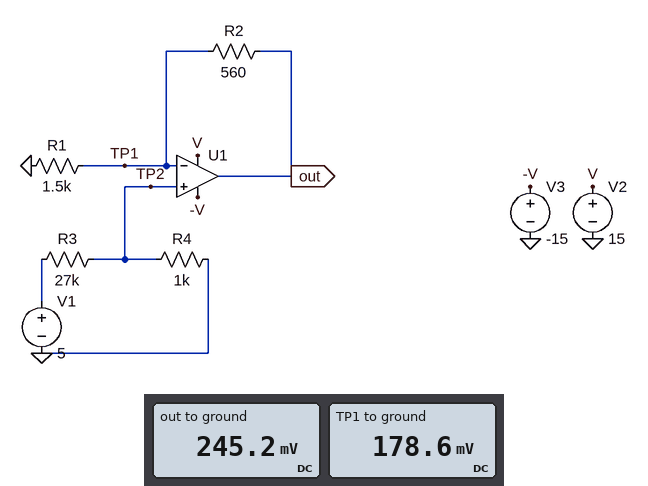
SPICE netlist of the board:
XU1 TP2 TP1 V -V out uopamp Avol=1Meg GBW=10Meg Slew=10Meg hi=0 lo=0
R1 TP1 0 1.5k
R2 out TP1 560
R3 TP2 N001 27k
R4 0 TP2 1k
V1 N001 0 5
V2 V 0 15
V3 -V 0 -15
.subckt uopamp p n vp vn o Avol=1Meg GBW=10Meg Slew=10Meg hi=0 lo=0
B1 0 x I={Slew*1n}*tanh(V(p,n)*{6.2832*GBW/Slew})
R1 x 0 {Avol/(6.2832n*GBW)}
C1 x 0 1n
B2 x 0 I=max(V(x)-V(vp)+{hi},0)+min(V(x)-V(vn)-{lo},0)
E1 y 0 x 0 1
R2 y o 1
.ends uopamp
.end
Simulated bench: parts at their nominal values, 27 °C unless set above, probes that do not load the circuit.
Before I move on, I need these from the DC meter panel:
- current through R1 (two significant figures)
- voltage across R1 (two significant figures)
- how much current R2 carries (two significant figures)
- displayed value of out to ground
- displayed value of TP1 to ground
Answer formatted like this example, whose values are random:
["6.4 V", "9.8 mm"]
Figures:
["120 µA", "180 mV", "120 µA", "245.2 mV", "178.6 mV"]
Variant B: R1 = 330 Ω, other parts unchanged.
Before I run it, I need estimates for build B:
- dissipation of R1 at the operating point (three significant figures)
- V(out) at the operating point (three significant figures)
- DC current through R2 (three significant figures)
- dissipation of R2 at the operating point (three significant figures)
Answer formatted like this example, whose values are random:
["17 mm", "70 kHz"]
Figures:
["96.6 µW", "482 mV", "541 µA", "164 µW"]
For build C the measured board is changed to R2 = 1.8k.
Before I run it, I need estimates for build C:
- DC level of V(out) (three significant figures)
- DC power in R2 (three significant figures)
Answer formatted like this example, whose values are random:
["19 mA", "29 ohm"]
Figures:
["393 mV", "25.5 µW"]
